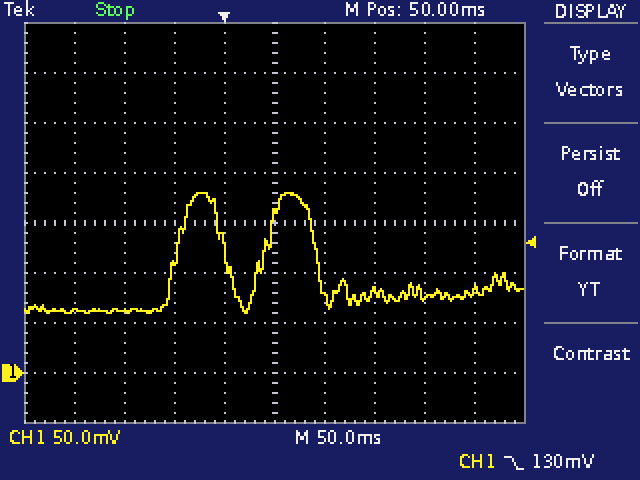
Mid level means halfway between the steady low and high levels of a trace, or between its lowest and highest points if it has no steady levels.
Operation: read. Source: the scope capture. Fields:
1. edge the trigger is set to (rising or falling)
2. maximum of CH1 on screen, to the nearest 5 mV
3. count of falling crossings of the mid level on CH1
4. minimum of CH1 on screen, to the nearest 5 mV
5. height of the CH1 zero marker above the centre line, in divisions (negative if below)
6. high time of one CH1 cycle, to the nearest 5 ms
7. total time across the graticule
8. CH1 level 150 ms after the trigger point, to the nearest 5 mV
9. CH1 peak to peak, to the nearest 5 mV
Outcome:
falling
180 mV
2
60 mV
-3.0 div
50 ms
500 ms
80 mV
120 mV
